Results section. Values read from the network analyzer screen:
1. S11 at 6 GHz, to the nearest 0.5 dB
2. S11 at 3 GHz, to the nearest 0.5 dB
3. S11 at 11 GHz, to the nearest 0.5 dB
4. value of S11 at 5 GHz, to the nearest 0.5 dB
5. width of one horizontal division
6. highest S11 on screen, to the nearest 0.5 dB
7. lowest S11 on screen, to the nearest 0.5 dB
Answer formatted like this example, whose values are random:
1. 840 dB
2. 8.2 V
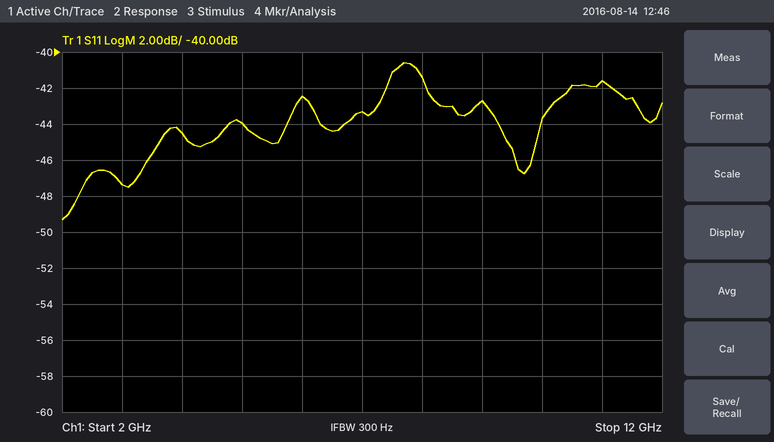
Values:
1. -42.5 dB
2. -47.5 dB
3. -41.5 dB
4. -44.0 dB
5. 1 GHz
6. -40.5 dB
7. -49.5 dB
